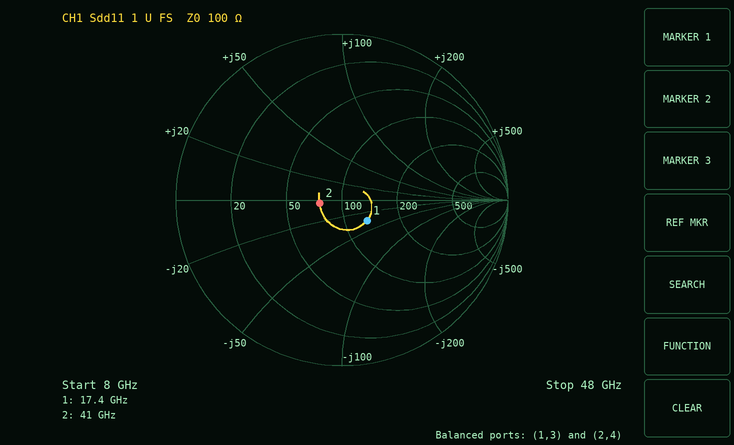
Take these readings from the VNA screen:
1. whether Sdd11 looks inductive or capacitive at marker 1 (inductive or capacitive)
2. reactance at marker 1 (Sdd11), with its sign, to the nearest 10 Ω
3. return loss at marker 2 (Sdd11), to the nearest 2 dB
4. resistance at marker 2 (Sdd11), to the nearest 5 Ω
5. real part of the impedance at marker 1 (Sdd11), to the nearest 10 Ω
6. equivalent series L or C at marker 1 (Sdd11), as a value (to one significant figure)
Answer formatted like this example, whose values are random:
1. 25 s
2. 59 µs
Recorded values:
1. capacitive
2. -30 Ω
3. 18 dB
4. 75 Ω
5. 130 Ω
6. 300 fF
